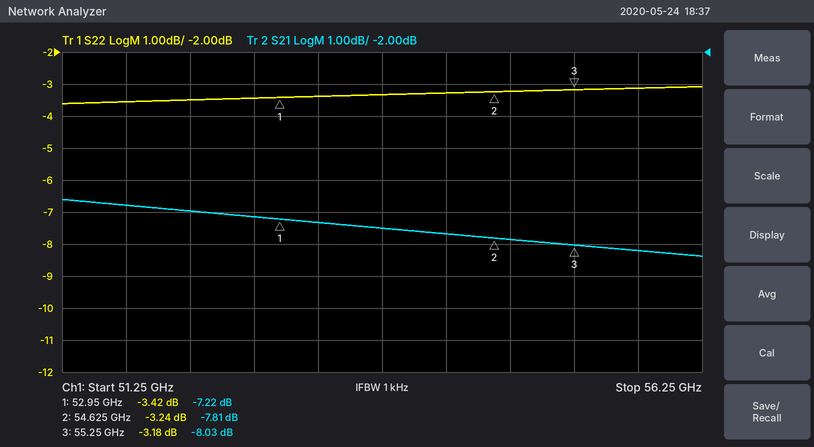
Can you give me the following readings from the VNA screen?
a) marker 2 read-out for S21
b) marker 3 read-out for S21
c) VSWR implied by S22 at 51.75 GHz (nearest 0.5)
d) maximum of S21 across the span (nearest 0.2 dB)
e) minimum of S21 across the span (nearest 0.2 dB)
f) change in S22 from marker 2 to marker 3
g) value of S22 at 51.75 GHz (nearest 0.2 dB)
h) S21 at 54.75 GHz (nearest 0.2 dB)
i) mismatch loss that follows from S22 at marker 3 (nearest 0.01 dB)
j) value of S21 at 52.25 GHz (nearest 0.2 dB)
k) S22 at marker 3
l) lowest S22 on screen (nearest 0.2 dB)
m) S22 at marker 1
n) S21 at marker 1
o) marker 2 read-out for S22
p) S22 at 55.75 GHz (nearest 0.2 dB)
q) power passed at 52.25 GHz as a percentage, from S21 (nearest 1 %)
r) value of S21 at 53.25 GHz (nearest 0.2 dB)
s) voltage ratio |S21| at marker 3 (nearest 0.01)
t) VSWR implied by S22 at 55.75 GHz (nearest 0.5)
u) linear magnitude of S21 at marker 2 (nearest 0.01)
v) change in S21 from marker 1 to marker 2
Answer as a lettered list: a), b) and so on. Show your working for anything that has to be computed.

a) -7.81 dB
b) -8.03 dB
c) |Γ| = 10^(-3.6/20) = 0.6607; VSWR = (1 + 0.6607)/(1 − 0.6607) ≈ 4.89, so 5.0 to the nearest 0.5
d) -6.6 dB
e) -8.4 dB
f) -3.18 − (-3.24) = 0.06 dB
g) -3.6 dB
h) -7.8 dB
i) −10 log10(1 − 10^(-3.18/10)) ≈ 2.85 dB
j) -7.0 dB
k) -3.18 dB
l) -3.6 dB
m) -3.42 dB
n) -7.22 dB
o) -3.24 dB
p) -3.2 dB
q) 10^(-7/10) ≈ 20 %
r) -7.4 dB
s) 10^(-8.03/20) ≈ 0.40
t) |Γ| = 10^(-3.2/20) = 0.6918; VSWR = (1 + 0.6918)/(1 − 0.6918) ≈ 5.5
u) 10^(-7.81/20) ≈ 0.41
v) -7.81 − (-7.22) = -0.59 dB
